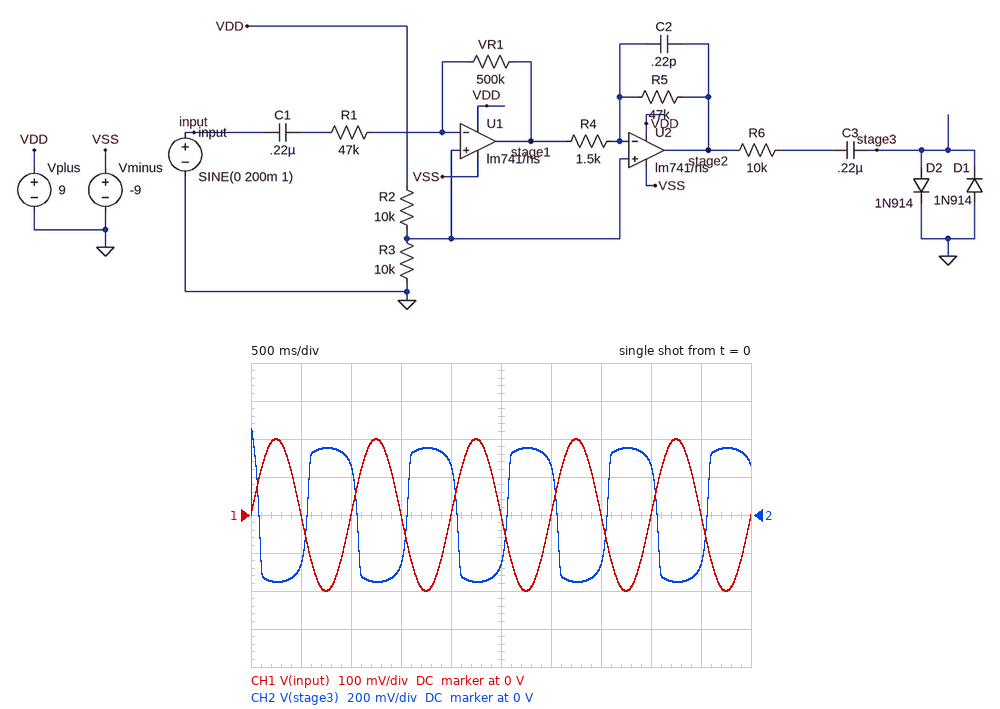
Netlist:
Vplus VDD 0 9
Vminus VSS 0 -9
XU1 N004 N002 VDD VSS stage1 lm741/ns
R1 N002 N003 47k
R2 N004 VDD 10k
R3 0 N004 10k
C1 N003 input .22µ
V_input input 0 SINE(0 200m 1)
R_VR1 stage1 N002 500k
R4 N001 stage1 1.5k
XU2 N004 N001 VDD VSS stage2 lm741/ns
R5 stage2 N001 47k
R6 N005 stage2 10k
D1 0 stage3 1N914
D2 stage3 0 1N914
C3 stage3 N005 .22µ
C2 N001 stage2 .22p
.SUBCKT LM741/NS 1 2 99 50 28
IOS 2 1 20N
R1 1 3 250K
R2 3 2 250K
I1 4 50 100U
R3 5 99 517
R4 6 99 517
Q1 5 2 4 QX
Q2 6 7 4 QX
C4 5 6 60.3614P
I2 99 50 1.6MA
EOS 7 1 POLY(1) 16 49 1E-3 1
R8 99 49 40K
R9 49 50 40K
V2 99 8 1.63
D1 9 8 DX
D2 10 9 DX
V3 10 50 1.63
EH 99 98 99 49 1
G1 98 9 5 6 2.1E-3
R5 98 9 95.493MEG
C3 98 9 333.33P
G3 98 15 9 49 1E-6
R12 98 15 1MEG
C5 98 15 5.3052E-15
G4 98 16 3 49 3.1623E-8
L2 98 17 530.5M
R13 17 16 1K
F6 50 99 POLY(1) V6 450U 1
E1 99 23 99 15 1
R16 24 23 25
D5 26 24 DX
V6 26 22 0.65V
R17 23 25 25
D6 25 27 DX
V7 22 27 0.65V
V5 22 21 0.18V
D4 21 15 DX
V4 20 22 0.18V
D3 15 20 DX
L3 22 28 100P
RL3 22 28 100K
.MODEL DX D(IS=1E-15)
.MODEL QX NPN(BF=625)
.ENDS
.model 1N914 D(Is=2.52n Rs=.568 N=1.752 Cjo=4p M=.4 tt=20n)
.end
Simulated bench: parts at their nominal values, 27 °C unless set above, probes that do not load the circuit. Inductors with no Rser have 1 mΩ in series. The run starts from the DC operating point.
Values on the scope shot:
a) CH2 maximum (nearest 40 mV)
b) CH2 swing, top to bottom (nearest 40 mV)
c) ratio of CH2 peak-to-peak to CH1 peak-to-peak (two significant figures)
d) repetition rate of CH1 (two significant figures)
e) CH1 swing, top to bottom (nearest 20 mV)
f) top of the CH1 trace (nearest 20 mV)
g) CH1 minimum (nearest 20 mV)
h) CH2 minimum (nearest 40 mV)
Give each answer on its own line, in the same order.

440 mV
800 mV
2.0
1.0 Hz
400 mV
200 mV
-200 mV
-360 mV
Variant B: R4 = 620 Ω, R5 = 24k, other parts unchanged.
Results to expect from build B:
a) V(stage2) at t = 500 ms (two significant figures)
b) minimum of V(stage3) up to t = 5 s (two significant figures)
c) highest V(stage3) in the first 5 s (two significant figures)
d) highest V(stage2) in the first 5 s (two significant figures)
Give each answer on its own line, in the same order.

-2.8 V
-360 mV
460 mV
7.9 V
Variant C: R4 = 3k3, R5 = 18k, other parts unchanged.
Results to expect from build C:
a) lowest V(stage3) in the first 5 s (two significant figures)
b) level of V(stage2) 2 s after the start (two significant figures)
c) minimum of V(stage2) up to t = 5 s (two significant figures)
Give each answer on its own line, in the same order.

-270 mV
5.0 V
3.5 V
